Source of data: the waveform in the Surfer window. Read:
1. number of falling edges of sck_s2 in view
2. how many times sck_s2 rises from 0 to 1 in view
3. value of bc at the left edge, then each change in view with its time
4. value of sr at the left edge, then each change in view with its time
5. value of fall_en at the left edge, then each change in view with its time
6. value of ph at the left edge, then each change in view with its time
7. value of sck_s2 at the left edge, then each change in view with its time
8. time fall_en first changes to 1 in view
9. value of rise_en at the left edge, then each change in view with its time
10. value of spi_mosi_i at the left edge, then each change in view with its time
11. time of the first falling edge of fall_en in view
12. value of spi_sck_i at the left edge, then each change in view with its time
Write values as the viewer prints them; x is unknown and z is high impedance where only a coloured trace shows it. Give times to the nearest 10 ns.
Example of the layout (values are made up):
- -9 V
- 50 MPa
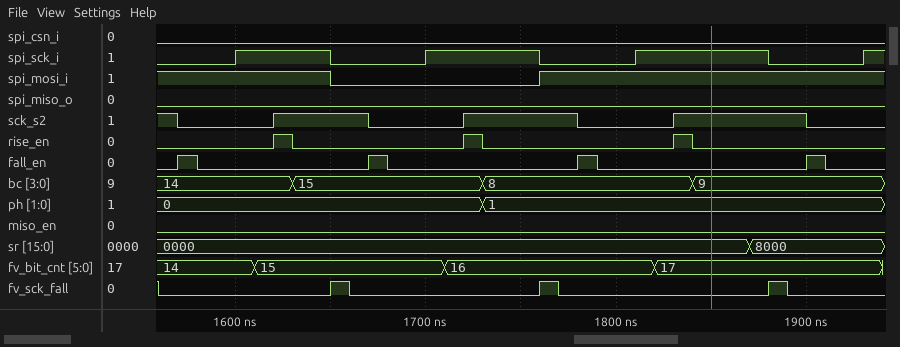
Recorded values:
- 4
- 3
- 14, 15 at 1630 ns, 8 at 1730 ns, 9 at 1840 ns
- 0000, 8000 at 1870 ns
- 0, 1 at 1570 ns, 0 at 1580 ns, 1 at 1670 ns, 0 at 1680 ns, 1 at 1780 ns, 0 at 1790 ns, 1 at 1900 ns, 0 at 1910 ns
- 0, 1 at 1730 ns
- 1, 0 at 1570 ns, 1 at 1620 ns, 0 at 1670 ns, 1 at 1720 ns, 0 at 1780 ns, 1 at 1830 ns, 0 at 1900 ns
- 1570 ns
- 0, 1 at 1620 ns, 0 at 1630 ns, 1 at 1720 ns, 0 at 1730 ns, 1 at 1830 ns, 0 at 1840 ns
- 1, 0 at 1650 ns, 1 at 1760 ns
- 1580 ns
- 0, 1 at 1600 ns, 0 at 1650 ns, 1 at 1700 ns, 0 at 1760 ns, 1 at 1810 ns, 0 at 1880 ns, 1 at 1930 ns
